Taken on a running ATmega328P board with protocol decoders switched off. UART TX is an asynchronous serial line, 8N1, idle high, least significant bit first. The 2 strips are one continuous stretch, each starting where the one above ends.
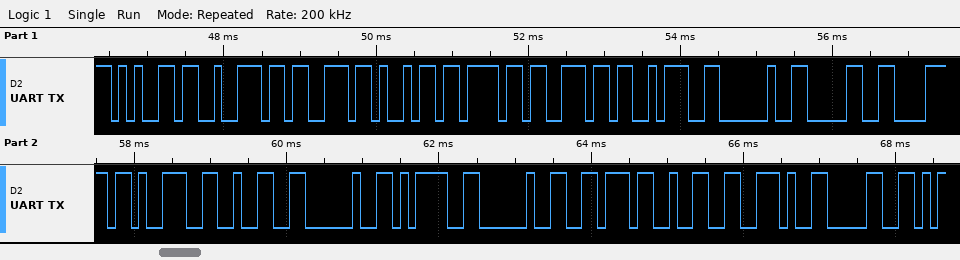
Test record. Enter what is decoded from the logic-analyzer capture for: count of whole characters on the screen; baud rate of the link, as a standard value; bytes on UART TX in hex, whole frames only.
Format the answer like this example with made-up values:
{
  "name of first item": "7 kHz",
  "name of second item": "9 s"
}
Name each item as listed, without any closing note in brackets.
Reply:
{
  "count of whole characters on the screen": "19",
  "baud rate of the link, as a standard value": "9600 baud",
  "bytes on UART TX in hex, whole frames only": "0x65 0x72 0x73 0x69 0x6F 0x6E 0x3A 0x20 0x30 0x78 0x39 0x32 0x20 0x3D 0x20 0x76 0x32 0x2E 0x30"
}
